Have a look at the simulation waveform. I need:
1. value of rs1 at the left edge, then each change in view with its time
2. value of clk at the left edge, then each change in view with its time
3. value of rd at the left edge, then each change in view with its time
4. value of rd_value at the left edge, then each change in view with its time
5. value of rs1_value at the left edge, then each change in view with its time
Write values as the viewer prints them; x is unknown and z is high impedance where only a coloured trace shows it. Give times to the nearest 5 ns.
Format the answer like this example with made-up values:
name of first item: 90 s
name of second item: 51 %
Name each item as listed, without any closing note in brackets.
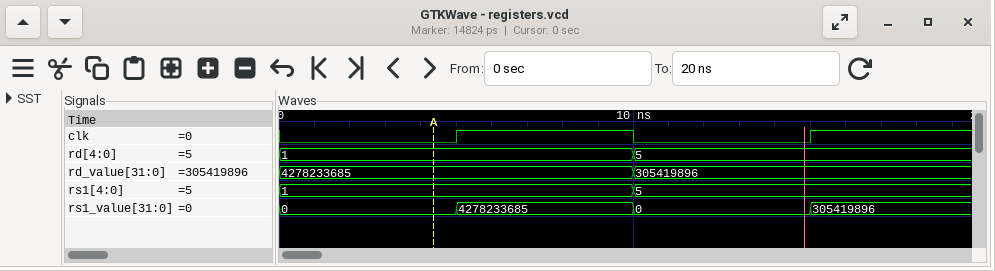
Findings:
value of rs1 at the left edge, then each change in view with its time: 1, 5 at 10 ns
value of clk at the left edge, then each change in view with its time: 0, 1 at 5 ns, 0 at 10 ns, 1 at 15 ns
value of rd at the left edge, then each change in view with its time: 1, 5 at 10 ns
value of rd_value at the left edge, then each change in view with its time: 4278233685, 305419896 at 10 ns
value of rs1_value at the left edge, then each change in view with its time: 0, 4278233685 at 5 ns, 0 at 10 ns, 305419896 at 15 ns
